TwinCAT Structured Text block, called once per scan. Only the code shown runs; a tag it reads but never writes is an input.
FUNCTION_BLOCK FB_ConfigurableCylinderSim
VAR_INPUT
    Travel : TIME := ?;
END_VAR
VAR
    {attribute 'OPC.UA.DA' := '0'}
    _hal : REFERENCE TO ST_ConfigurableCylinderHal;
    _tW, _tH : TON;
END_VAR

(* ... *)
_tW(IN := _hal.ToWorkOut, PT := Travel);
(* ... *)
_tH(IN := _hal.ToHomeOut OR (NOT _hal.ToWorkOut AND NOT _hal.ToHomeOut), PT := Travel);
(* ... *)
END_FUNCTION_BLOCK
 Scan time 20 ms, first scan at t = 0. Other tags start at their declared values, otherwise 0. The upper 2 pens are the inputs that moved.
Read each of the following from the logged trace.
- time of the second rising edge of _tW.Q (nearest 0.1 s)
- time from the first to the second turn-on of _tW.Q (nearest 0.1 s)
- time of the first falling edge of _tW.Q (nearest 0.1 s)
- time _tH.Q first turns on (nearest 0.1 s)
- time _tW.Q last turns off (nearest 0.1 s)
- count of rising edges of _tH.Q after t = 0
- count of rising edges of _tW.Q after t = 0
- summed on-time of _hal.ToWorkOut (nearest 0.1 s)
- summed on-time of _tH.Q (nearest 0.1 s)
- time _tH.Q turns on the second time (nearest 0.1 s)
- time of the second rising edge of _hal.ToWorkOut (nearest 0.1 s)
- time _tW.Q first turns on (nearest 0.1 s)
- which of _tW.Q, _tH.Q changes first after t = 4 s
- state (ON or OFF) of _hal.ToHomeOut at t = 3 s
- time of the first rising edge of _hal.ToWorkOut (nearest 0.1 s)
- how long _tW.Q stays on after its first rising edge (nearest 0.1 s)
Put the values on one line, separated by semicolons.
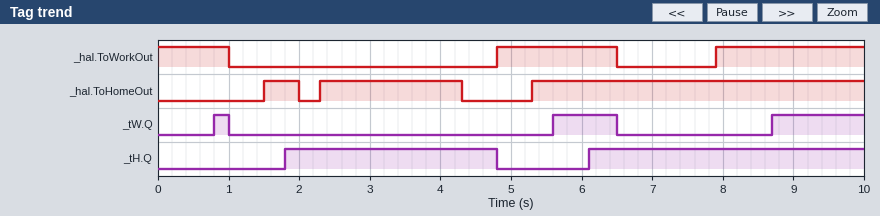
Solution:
5.6 s; 4.8 s; 1.0 s; 1.8 s; 6.5 s; 2; 3; 4.8 s; 6.9 s; 6.1 s; 7.9 s; 0.8 s; _tH.Q; ON; 4.8 s; 0.2 s
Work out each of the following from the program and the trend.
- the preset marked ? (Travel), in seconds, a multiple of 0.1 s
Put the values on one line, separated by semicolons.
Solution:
0.8 s
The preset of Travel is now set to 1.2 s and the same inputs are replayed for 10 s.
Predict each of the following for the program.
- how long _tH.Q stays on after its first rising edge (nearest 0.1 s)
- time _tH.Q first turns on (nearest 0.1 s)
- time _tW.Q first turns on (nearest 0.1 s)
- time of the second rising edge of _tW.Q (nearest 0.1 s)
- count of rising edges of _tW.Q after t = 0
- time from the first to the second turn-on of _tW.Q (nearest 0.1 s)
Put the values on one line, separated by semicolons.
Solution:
2.6 s; 2.2 s; 6.0 s; 9.1 s; 2; 3.1 s
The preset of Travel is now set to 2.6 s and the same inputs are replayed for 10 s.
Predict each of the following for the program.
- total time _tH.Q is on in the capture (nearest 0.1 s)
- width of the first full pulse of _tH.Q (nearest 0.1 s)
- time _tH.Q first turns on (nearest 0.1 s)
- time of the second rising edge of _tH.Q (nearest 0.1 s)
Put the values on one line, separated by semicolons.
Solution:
3.3 s; 1.2 s; 3.6 s; 7.9 s
